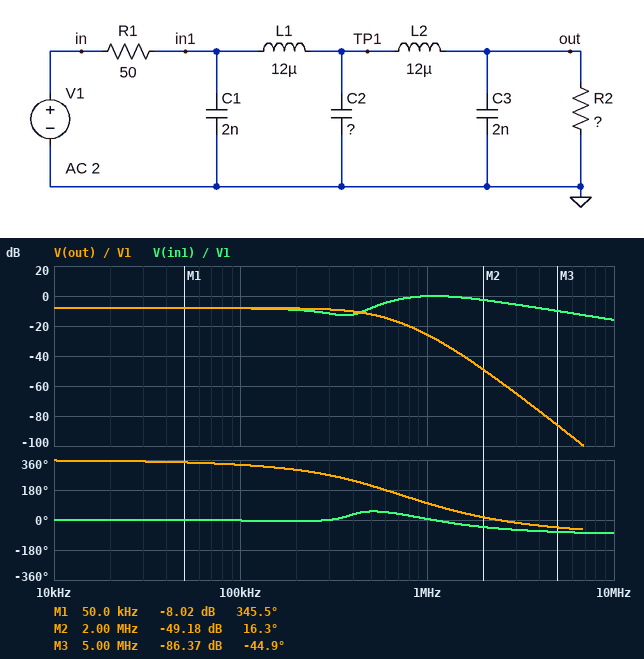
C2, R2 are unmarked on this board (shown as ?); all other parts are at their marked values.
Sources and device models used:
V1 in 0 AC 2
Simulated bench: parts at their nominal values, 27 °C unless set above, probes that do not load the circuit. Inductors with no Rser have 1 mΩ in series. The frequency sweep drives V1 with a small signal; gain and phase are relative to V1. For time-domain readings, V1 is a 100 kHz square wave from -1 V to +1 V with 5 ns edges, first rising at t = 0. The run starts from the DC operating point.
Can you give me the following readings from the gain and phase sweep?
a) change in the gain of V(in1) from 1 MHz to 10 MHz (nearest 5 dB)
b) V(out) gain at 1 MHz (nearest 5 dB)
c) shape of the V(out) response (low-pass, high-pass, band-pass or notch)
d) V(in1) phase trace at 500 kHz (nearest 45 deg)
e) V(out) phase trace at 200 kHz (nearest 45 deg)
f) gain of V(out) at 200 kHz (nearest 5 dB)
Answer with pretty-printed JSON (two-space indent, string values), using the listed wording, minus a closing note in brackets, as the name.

{
  "change in the gain of V(in1) from 1 MHz to 10 MHz": "-15 dB",
  "V(out) gain at 1 MHz": "-25 dB",
  "shape of the V(out) response": "low-pass",
  "V(in1) phase trace at 500 kHz": "45 deg",
  "V(out) phase trace at 200 kHz": "315 deg",
  "gain of V(out) at 200 kHz": "-10 dB"
}
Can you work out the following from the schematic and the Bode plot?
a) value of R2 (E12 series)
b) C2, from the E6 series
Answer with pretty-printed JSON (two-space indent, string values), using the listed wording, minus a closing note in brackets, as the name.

{
  "value of R2": "33 Ω",
  "C2, from the E6 series": "22 nF"
}
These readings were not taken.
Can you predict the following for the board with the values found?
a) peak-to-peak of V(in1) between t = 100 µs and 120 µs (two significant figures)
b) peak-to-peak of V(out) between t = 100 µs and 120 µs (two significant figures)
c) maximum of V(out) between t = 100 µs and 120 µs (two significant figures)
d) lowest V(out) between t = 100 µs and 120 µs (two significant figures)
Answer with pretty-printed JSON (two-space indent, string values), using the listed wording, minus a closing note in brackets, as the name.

{
  "peak-to-peak of V(in1) between t = 100 µs and 120 µs": "1.9 V",
  "peak-to-peak of V(out) between t = 100 µs and 120 µs": "860 mV",
  "maximum of V(out) between t = 100 µs and 120 µs": "430 mV",
  "lowest V(out) between t = 100 µs and 120 µs": "-430 mV"
}
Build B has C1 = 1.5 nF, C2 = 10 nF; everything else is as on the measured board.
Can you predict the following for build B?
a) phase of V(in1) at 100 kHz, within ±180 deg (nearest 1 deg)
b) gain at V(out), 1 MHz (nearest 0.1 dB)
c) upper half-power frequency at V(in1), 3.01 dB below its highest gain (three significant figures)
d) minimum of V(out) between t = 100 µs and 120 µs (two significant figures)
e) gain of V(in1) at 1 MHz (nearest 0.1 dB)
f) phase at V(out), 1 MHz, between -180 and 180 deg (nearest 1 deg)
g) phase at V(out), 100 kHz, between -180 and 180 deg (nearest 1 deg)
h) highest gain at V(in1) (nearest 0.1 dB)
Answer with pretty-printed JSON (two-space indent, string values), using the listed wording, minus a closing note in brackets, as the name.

{
  "phase of V(in1) at 100 kHz, within ±180 deg": "5 deg",
  "gain at V(out), 1 MHz": "-17.1 dB",
  "upper half-power frequency at V(in1), 3.01 dB below its highest gain": "2.68 MHz",
  "minimum of V(out) between t = 100 µs and 120 µs": "-490 mV",
  "gain of V(in1) at 1 MHz": "-1.0 dB",
  "phase at V(out), 1 MHz, between -180 and 180 deg": "123 deg",
  "phase at V(out), 100 kHz, between -180 and 180 deg": "-20 deg",
  "highest gain at V(in1)": "0 dB"
}
